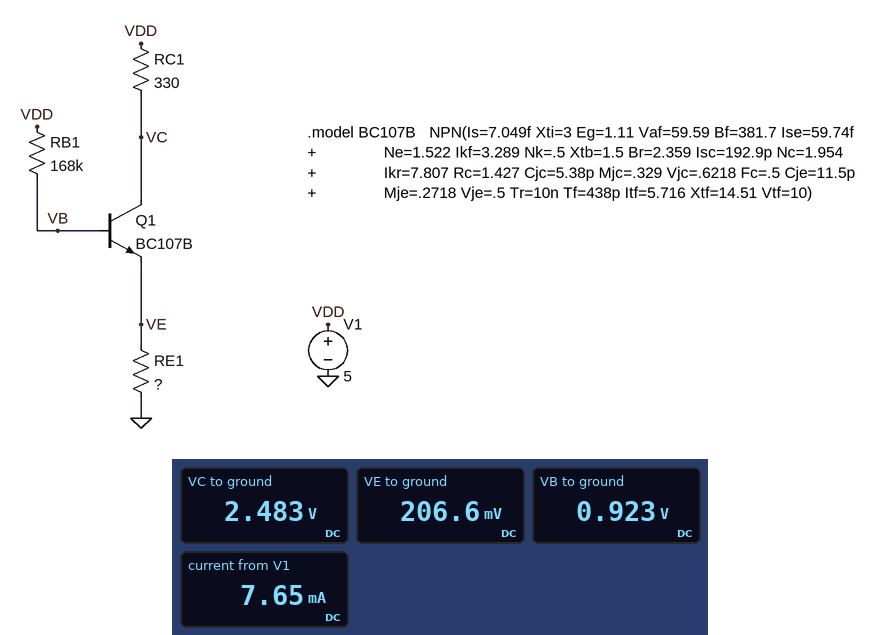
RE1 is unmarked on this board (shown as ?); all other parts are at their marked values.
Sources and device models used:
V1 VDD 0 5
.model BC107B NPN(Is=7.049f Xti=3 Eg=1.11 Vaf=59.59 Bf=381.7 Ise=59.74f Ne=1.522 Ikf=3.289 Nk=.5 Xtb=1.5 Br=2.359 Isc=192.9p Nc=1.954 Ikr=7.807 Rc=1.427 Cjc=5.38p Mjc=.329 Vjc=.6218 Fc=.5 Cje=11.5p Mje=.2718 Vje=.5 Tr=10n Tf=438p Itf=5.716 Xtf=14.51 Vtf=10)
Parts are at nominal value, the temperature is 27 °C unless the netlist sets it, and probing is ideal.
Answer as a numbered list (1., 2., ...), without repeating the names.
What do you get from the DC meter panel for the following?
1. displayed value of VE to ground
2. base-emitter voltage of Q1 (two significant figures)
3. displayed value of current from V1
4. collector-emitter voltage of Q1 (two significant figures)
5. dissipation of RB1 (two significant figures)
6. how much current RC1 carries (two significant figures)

1. 206.6 mV
2. 720 mV
3. 7.65 mA
4. 2.3 V
5. 99 µW
6. 7.6 mA
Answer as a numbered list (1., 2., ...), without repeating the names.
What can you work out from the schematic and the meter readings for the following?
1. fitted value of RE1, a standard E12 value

1. 27 Ω
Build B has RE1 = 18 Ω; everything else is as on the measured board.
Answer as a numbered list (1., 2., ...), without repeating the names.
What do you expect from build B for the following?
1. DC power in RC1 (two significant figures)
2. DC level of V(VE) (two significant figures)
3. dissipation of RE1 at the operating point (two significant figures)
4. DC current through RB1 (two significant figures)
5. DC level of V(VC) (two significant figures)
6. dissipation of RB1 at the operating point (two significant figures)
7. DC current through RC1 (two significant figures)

1. 20 mW
2. 140 mV
3. 1.1 mW
4. 25 µA
5. 2.4 V
6. 100 µW
7. 7.8 mA
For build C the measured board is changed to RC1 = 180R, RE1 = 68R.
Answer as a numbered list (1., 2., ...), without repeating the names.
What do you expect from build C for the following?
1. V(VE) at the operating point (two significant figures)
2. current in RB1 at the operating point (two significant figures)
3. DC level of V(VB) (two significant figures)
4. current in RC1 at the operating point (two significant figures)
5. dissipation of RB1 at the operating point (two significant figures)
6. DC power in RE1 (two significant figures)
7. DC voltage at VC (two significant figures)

1. 490 mV
2. 23 µA
3. 1.2 V
4. 7.2 mA
5. 86 µW
6. 3.5 mW
7. 3.7 V
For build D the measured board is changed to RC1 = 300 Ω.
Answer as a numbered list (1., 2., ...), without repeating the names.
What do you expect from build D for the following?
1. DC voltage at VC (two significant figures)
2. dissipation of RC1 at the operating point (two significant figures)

1. 2.7 V
2. 18 mW
